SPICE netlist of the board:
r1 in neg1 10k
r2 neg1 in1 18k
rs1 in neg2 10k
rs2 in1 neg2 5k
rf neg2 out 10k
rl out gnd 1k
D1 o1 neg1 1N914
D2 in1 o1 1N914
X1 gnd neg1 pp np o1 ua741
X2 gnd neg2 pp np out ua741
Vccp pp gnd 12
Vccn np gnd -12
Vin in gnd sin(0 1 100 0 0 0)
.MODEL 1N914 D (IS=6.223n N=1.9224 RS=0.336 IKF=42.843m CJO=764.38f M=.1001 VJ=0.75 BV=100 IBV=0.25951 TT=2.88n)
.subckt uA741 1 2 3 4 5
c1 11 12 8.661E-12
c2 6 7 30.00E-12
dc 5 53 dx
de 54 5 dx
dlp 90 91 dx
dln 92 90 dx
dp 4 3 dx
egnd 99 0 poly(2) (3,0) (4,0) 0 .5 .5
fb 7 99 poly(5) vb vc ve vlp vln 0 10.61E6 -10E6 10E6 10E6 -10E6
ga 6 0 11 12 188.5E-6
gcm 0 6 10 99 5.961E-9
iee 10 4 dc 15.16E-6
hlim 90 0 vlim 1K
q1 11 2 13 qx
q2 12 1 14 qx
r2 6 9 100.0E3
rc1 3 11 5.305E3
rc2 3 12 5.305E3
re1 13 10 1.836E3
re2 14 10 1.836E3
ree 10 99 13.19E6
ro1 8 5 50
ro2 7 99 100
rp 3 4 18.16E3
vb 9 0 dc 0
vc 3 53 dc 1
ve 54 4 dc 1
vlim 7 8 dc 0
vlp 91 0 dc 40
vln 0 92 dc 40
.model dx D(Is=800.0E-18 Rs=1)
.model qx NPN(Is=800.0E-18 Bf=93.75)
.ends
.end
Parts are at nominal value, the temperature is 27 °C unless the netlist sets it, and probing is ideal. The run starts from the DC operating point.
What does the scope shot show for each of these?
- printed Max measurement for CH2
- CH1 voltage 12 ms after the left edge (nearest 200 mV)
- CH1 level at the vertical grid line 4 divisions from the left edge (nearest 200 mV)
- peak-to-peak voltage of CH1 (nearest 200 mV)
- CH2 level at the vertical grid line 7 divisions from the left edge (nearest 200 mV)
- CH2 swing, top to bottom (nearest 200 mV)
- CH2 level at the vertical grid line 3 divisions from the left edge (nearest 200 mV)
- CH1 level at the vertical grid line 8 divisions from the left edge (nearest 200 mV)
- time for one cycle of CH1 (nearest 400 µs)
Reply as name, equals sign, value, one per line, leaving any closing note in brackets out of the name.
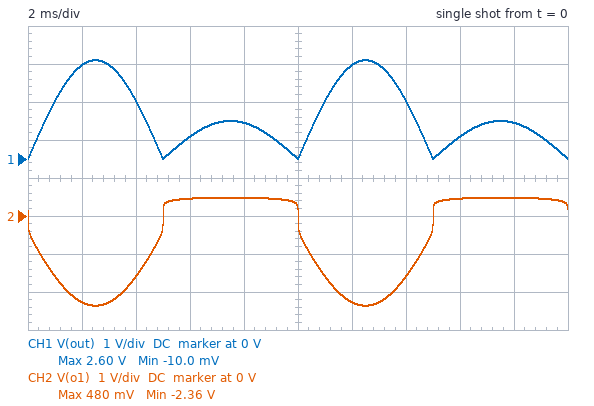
printed Max measurement for CH2 = 480 mV
CH1 voltage 12 ms after the left edge = 2.4 V
CH1 level at the vertical grid line 4 divisions from the left edge = 1.0 V
peak-to-peak voltage of CH1 = 2.6 V
CH2 level at the vertical grid line 7 divisions from the left edge = -1.6 V
CH2 swing, top to bottom = 2.8 V
CH2 level at the vertical grid line 3 divisions from the left edge = 400 mV
CH1 level at the vertical grid line 8 divisions from the left edge = 600 mV
time for one cycle of CH1 = 10.0 ms
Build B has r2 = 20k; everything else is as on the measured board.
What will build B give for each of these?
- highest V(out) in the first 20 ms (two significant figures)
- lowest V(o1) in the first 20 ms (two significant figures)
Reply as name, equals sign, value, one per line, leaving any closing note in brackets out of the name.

highest V(out) in the first 20 ms = 3.0 V
lowest V(o1) in the first 20 ms = -2.6 V
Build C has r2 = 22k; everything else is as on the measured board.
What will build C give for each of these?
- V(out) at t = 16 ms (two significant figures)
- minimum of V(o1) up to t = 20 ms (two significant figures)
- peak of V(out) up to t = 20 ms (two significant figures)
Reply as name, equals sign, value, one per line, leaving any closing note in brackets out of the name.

V(out) at t = 16 ms = 590 mV
minimum of V(o1) up to t = 20 ms = -2.8 V
peak of V(out) up to t = 20 ms = 3.4 V
